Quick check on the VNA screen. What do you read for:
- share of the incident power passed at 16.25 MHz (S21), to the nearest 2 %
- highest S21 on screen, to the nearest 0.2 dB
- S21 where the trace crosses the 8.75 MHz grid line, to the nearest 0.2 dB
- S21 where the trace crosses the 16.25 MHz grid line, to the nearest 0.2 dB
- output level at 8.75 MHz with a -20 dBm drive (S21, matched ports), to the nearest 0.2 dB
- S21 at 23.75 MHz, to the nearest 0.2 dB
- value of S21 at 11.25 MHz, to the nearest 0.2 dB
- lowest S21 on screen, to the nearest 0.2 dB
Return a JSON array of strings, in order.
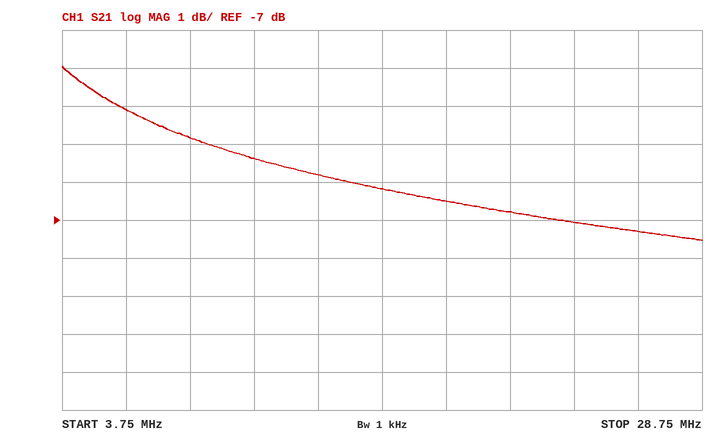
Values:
["24 %", "-3.0 dB", "-4.8 dB", "-6.2 dB", "-24.8 dBm", "-7.0 dB", "-5.4 dB", "-7.6 dB"]
